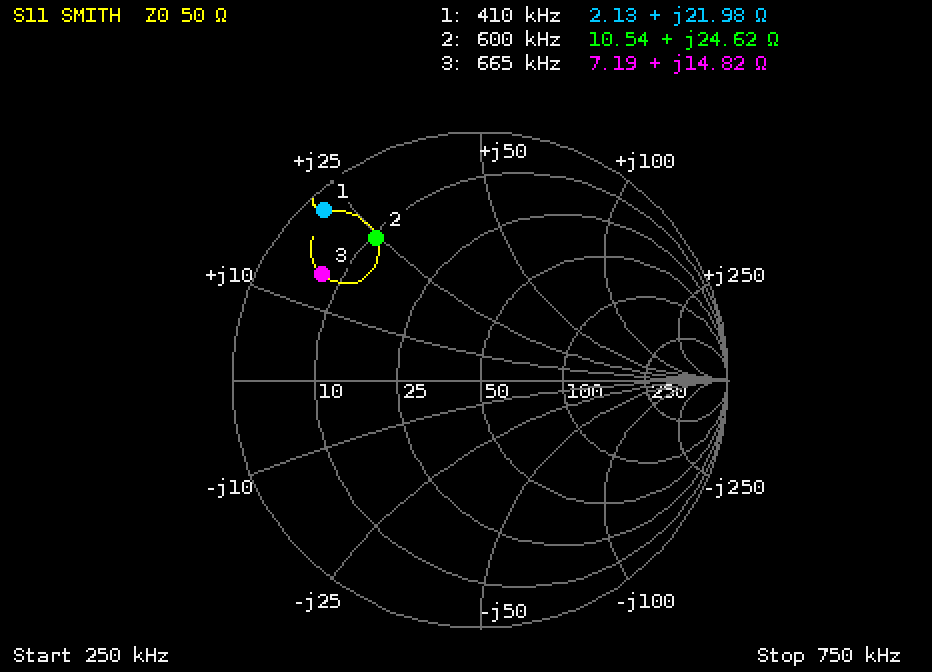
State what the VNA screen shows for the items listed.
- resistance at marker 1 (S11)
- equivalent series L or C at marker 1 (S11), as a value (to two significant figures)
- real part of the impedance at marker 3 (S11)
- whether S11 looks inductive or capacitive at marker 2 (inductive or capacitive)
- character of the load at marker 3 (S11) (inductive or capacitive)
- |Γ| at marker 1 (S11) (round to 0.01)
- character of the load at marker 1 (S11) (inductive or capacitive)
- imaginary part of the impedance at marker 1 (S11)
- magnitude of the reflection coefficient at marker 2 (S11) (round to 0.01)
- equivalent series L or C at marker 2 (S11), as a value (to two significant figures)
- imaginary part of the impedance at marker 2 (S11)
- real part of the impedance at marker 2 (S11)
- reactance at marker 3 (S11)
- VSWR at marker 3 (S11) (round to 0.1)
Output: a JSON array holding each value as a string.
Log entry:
["2.13 Ω", "8.5 µH", "7.19 Ω", "inductive", "inductive", "0.93", "inductive", "+21.98 Ω", "0.71", "6.5 µH", "+24.62 Ω", "10.54 Ω", "+14.82 Ω", "7.6"]
